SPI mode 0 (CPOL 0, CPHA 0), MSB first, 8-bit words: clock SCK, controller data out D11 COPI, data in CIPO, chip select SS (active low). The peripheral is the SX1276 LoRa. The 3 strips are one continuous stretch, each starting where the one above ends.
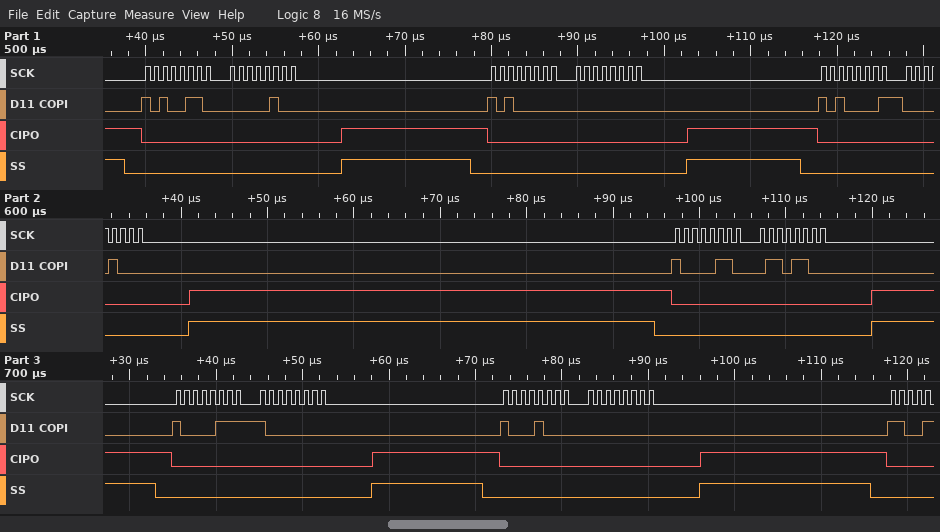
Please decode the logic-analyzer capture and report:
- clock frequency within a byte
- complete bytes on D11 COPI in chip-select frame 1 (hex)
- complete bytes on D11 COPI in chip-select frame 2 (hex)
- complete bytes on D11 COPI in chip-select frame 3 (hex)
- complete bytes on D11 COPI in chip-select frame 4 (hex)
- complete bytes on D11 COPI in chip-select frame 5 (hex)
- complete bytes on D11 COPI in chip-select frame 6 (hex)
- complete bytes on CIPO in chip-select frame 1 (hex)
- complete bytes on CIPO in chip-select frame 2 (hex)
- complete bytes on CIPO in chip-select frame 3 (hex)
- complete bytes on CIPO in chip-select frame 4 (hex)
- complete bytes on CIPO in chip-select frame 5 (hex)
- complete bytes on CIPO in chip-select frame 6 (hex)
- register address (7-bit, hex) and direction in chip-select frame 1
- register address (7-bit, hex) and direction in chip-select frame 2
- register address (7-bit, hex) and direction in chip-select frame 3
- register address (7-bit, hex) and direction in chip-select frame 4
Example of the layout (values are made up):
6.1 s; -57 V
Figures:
1 MHz; A6 04; A0 00; A1 08; 86 6C; 87 80; 88 00; 00 00; 00 00; 00 00; 00 00; 00 00; 00 00; 0x26 write; 0x20 write; 0x21 write; 0x06 write
